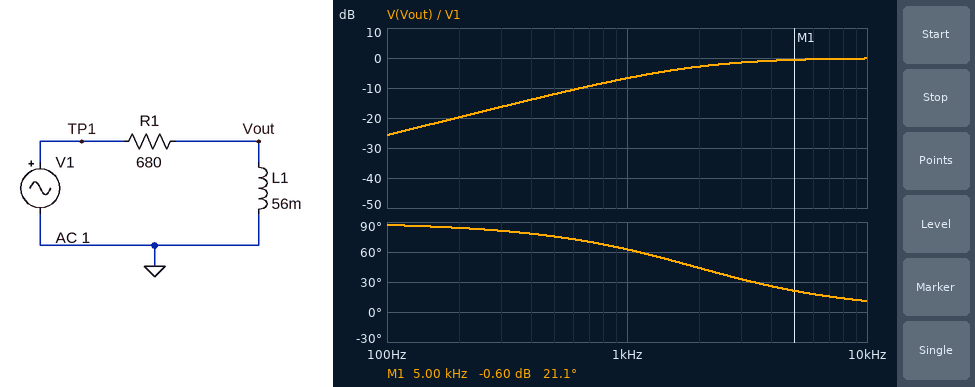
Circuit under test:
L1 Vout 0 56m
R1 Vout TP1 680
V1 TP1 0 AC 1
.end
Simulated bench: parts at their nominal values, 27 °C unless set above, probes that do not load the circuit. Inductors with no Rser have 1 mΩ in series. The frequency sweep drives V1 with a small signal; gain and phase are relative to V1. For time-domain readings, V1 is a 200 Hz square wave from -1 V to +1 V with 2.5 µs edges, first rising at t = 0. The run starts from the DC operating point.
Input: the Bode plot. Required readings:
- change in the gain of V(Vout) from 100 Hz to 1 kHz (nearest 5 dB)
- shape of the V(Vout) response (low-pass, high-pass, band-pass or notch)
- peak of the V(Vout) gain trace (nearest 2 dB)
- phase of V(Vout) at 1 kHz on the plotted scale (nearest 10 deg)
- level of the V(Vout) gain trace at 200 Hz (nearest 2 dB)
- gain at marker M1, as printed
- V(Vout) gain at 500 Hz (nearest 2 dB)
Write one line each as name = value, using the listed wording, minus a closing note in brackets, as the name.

change in the gain of V(Vout) from 100 Hz to 1 kHz = 20 dB
shape of the V(Vout) response = high-pass
peak of the V(Vout) gain trace = 0 dB
phase of V(Vout) at 1 kHz on the plotted scale = 60 deg
level of the V(Vout) gain trace at 200 Hz = -20 dB
gain at marker M1, as printed = -0.60 dB
V(Vout) gain at 500 Hz = -12 dB
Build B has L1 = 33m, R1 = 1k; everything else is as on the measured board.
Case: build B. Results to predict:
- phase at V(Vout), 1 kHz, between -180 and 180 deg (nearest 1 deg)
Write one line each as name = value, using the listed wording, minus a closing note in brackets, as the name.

phase at V(Vout), 1 kHz, between -180 and 180 deg = 78 deg
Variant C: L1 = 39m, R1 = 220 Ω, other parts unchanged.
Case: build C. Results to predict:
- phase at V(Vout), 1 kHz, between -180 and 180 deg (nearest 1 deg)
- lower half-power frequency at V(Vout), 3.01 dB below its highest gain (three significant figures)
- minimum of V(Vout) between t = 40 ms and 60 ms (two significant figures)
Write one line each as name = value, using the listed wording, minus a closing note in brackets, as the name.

phase at V(Vout), 1 kHz, between -180 and 180 deg = 42 deg
lower half-power frequency at V(Vout), 3.01 dB below its highest gain = 898 Hz
minimum of V(Vout) between t = 40 ms and 60 ms = -2.0 V
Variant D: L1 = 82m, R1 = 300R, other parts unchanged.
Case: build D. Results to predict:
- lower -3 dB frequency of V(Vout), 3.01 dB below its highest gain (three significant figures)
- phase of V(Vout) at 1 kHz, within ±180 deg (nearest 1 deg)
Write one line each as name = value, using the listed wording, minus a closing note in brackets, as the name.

lower -3 dB frequency of V(Vout), 3.01 dB below its highest gain = 582 Hz
phase of V(Vout) at 1 kHz, within ±180 deg = 30 deg
